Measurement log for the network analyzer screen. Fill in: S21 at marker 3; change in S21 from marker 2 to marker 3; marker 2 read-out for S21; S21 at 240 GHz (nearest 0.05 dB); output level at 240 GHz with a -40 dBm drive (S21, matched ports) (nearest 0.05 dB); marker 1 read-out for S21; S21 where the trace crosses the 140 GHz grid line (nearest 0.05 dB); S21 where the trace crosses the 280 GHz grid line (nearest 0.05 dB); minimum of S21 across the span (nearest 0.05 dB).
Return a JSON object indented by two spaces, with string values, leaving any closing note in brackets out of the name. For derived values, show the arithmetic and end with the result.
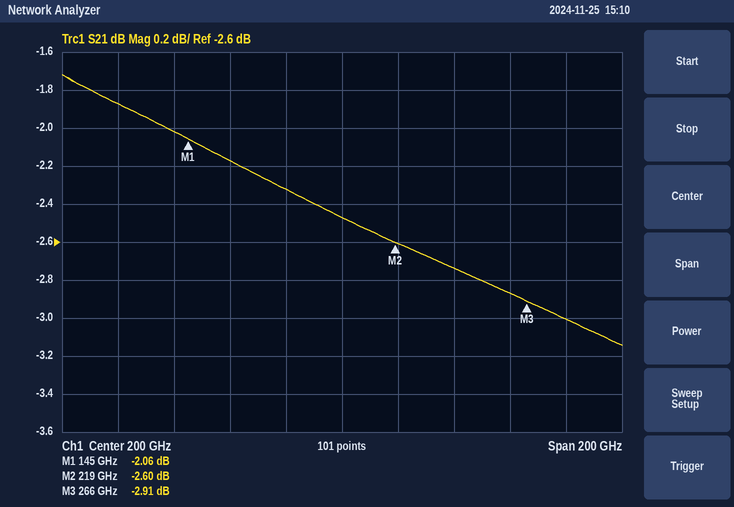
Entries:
{
  "S21 at marker 3": "-2.91 dB",
  "change in S21 from marker 2 to marker 3": "-2.91 − (-2.6) = -0.31 dB",
  "marker 2 read-out for S21": "-2.60 dB",
  "S21 at 240 GHz": "-2.75 dB",
  "output level at 240 GHz with a -40 dBm drive (S21, matched ports)": "-40 dBm + (-2.75 dB) = -42.75 dBm",
  "marker 1 read-out for S21": "-2.06 dB",
  "S21 where the trace crosses the 140 GHz grid line": "-2.00 dB",
  "S21 where the trace crosses the 280 GHz grid line": "-3.00 dB",
  "minimum of S21 across the span": "-3.15 dB"
}
